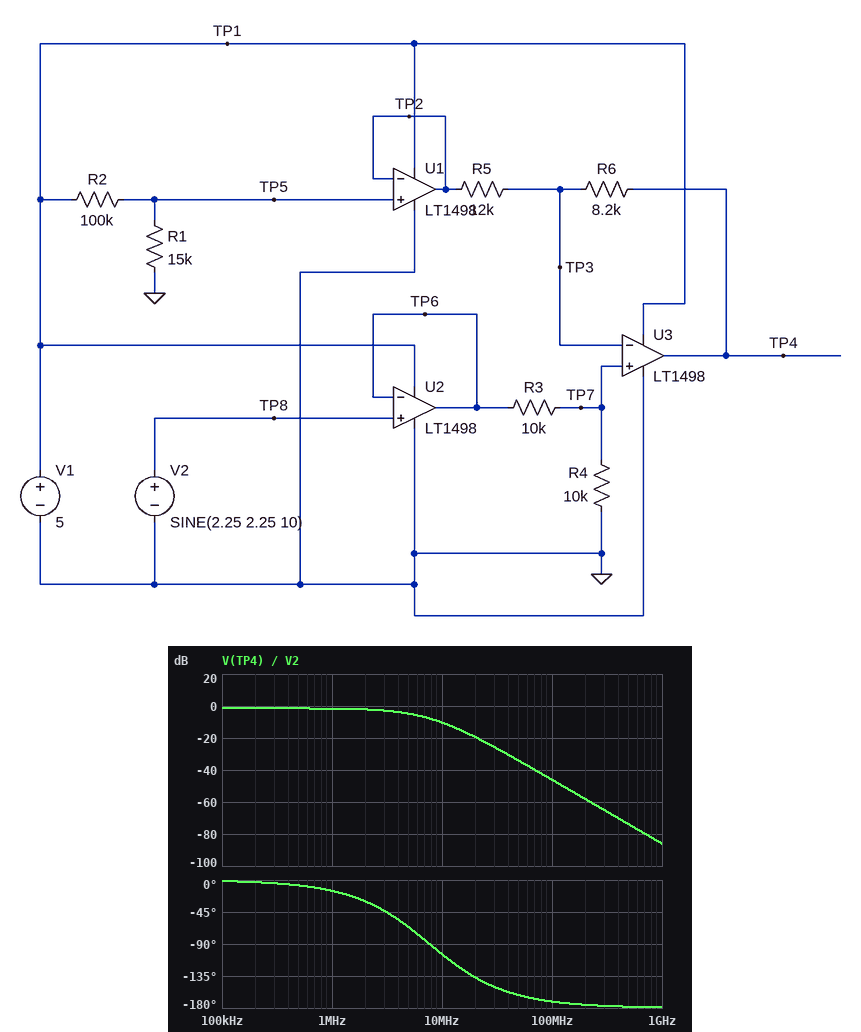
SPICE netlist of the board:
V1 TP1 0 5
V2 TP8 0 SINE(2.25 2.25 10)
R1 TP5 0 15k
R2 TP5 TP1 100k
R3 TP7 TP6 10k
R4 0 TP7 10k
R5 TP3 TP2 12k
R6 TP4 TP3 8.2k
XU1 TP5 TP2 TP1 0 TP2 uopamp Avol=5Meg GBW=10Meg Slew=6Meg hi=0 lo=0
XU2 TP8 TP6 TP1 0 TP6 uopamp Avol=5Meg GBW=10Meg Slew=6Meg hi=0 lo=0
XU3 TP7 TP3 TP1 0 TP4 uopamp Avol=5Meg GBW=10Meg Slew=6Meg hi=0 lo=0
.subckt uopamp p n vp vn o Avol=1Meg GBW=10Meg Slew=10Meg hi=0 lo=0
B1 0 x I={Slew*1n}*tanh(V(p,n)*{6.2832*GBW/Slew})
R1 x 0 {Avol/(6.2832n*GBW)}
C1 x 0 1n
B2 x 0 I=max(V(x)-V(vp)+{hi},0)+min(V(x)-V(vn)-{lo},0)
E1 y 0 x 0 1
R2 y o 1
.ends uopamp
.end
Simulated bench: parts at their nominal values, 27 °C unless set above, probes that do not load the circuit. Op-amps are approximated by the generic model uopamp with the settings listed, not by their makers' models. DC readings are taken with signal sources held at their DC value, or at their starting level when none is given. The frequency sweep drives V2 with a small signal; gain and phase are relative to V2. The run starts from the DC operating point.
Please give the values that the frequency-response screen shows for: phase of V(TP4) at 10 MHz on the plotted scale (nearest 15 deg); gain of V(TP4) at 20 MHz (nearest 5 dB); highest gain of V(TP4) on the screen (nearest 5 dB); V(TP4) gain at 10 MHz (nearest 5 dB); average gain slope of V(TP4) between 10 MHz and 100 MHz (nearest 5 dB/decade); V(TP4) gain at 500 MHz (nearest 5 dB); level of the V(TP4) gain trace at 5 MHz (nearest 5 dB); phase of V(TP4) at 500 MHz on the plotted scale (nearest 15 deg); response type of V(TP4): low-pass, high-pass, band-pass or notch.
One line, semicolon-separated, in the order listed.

-105 deg; -20 dB; 0 dB; -10 dB; -35 dB/decade; -75 dB; -5 dB; -180 deg; low-pass
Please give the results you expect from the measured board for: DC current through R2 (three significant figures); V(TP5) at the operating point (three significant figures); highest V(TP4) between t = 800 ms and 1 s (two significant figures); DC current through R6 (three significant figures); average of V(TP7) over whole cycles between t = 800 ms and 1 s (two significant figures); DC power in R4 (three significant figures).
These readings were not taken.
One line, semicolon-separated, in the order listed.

43.5 µA; 652 mV; 3.3 V; 39.4 µA; 1.1 V; 127 µW
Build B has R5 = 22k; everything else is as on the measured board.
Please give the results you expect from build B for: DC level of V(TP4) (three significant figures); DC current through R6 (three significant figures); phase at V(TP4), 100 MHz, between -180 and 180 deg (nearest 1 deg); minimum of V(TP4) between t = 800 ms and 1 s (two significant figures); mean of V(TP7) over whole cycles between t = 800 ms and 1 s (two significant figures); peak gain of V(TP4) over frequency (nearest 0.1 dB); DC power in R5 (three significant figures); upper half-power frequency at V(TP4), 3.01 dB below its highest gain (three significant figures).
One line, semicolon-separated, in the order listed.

1.30 V; 21.5 µA; -170 deg; -5.7 mV; 1.1 V; -3.3 dB; 10.2 µW; 5.40 MHz
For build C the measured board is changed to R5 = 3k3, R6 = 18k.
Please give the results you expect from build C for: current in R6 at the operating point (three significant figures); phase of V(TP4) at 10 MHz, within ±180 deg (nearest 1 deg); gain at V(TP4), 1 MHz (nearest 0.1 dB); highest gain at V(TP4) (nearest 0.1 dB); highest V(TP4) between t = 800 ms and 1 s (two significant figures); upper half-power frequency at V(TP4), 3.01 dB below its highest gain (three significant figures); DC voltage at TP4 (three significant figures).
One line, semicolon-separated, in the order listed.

143 µA; -126 deg; 8.6 dB; 10.2 dB; 5.0 V; 1.51 MHz; 3.70 V
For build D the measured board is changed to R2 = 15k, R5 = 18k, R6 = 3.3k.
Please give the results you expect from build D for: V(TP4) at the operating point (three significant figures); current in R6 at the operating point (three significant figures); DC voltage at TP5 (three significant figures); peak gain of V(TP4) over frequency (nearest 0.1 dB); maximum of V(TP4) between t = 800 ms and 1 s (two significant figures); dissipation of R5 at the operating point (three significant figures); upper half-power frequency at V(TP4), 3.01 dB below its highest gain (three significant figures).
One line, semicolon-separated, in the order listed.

873 mV; 76.4 µA; 2.50 V; -4.6 dB; 2.2 V; 105 µW; 5.89 MHz
